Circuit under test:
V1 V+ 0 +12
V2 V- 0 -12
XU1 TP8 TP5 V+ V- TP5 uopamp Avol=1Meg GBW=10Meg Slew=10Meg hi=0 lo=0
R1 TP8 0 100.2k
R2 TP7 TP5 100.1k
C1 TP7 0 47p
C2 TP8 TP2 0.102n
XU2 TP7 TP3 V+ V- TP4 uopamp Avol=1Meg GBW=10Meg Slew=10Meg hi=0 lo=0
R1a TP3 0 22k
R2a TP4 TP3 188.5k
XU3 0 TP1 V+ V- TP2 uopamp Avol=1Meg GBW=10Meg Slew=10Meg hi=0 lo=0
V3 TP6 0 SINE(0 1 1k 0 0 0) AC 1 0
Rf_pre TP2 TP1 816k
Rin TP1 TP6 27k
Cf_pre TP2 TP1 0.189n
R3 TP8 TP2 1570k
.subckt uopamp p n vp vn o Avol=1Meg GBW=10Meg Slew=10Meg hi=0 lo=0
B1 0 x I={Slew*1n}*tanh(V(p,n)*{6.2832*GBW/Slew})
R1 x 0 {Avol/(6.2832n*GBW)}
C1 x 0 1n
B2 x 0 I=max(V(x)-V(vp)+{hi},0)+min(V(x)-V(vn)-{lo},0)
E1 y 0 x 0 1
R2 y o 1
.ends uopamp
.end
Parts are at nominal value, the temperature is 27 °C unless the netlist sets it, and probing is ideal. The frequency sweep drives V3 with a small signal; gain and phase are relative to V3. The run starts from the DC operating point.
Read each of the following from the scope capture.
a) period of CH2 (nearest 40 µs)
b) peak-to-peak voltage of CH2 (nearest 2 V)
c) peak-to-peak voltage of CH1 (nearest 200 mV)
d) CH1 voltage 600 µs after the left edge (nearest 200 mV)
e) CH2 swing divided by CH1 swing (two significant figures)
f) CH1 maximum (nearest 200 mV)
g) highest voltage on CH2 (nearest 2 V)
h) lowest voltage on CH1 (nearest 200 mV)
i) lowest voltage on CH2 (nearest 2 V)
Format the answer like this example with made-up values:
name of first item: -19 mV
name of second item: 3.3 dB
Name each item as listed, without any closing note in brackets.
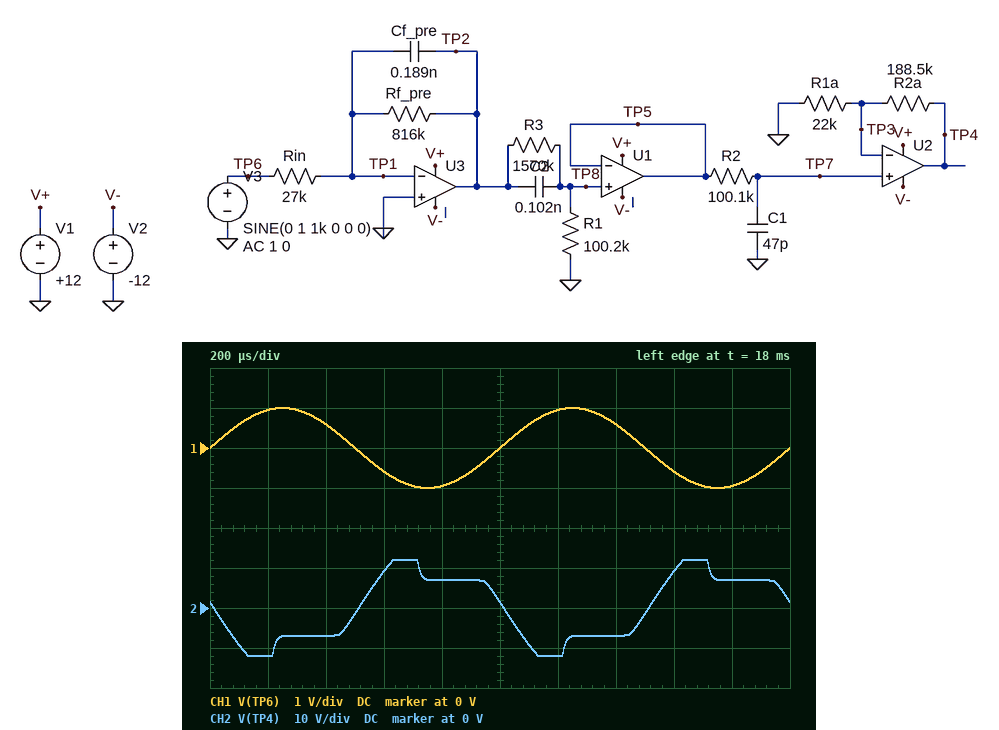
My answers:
period of CH2: 1.00 ms
peak-to-peak voltage of CH2: 24 V
peak-to-peak voltage of CH1: 2.0 V
CH1 voltage 600 µs after the left edge: -600 mV
CH2 swing divided by CH1 swing: 12
CH1 maximum: 1.0 V
highest voltage on CH2: 12 V
lowest voltage on CH1: -1.0 V
lowest voltage on CH2: -12 V
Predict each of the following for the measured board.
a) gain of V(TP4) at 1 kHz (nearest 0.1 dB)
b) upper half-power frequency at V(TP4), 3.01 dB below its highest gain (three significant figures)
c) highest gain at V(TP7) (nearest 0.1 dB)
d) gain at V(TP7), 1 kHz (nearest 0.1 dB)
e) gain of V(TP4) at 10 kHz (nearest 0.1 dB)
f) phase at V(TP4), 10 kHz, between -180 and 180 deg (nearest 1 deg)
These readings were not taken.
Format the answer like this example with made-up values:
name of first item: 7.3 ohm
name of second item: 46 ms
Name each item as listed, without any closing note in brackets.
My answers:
gain of V(TP4) at 1 kHz: 24.9 dB
upper half-power frequency at V(TP4), 3.01 dB below its highest gain: 14.3 kHz
highest gain at V(TP7): 5.3 dB
gain at V(TP7), 1 kHz: 5.3 dB
gain of V(TP4) at 10 kHz: 23.4 dB
phase at V(TP4), 10 kHz, between -180 and 180 deg: 132 deg
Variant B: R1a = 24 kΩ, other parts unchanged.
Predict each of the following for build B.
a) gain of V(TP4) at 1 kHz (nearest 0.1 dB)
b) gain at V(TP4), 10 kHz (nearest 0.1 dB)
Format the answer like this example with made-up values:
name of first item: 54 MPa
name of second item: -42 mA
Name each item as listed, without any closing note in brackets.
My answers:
gain of V(TP4) at 1 kHz: 24.2 dB
gain at V(TP4), 10 kHz: 22.7 dB
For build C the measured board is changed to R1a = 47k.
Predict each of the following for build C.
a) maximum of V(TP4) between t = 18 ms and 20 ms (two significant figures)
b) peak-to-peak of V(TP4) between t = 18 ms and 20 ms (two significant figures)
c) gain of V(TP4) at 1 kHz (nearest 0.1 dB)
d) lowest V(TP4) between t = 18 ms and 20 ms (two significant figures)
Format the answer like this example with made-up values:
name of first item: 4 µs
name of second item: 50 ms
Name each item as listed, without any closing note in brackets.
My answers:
maximum of V(TP4) between t = 18 ms and 20 ms: 8.6 V
peak-to-peak of V(TP4) between t = 18 ms and 20 ms: 17 V
gain of V(TP4) at 1 kHz: 19.3 dB
lowest V(TP4) between t = 18 ms and 20 ms: -8.6 V
